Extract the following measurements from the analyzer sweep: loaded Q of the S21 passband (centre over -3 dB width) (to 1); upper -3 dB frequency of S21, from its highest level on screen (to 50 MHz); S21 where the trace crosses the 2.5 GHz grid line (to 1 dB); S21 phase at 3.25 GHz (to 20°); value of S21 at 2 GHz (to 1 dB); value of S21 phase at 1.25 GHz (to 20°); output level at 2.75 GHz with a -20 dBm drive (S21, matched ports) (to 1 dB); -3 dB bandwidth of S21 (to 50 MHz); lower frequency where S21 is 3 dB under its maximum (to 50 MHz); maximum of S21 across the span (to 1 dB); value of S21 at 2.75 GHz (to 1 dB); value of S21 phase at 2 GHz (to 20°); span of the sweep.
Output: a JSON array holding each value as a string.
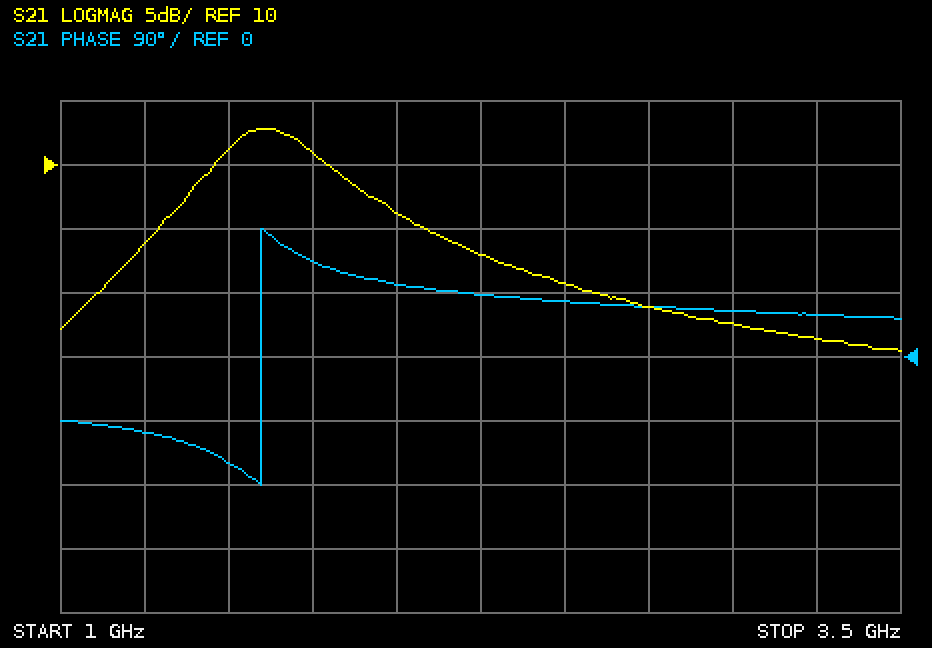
["5", "1.80 GHz", "1 dB", "60°", "6 dB", "-100°", "-21 dBm", "350 MHz", "1.45 GHz", "13 dB", "-1 dB", "100°", "2.5 GHz"]
